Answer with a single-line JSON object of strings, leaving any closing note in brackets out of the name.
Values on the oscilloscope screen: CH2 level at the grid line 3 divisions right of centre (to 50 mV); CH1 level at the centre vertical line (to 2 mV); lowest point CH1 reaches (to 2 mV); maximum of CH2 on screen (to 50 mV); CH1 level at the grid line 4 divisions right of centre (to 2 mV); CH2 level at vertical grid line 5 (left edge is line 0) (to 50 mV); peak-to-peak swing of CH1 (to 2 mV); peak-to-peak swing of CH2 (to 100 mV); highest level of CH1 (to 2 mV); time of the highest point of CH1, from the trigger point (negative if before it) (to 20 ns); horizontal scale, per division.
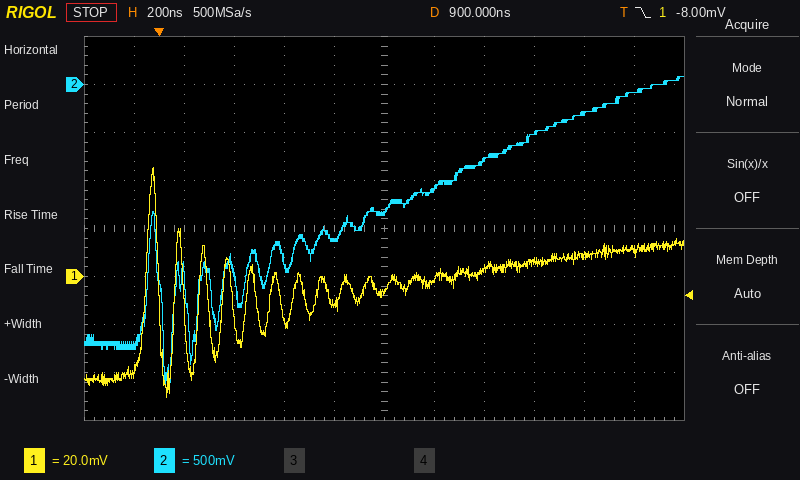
{"CH2 level at the grid line 3 divisions right of centre": "-500 mV", "CH1 level at the centre vertical line": "-6 mV", "lowest point CH1 reaches": "-50 mV", "maximum of CH2 on screen": "100 mV", "CH1 level at the grid line 4 divisions right of centre": "8 mV", "CH2 level at vertical grid line 5 (left edge is line 0)": "-1.60 V", "peak-to-peak swing of CH1": "96 mV", "peak-to-peak swing of CH2": "3.20 V", "highest level of CH1": "46 mV", "time of the highest point of CH1, from the trigger point (negative if before it)": "-20 ns", "horizontal scale, per division": "200 ns"}
